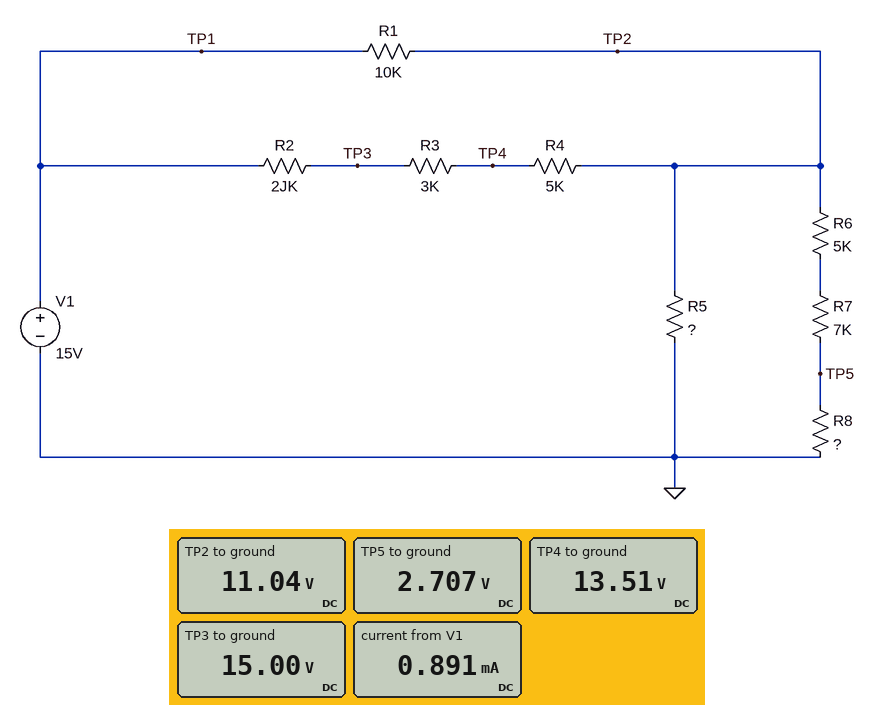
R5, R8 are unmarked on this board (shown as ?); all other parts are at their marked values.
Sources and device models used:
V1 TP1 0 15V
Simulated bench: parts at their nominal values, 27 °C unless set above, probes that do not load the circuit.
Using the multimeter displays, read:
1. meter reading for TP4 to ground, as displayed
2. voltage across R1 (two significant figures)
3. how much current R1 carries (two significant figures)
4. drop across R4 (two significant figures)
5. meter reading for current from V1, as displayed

13.51 V
4.0 V
400 µA
2.5 V
0.891 mA
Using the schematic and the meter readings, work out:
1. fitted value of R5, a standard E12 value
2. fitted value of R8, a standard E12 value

56 kΩ
3.9 kΩ
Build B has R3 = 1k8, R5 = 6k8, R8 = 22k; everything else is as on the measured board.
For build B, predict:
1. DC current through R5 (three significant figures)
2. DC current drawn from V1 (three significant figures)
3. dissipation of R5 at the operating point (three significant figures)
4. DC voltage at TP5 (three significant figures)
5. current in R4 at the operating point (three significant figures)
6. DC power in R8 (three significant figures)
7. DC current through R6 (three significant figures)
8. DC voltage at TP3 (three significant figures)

1.29 mA
1.54 mA
11.3 mW
5.66 V
919 µA
1.46 mW
257 µA
15.0 V
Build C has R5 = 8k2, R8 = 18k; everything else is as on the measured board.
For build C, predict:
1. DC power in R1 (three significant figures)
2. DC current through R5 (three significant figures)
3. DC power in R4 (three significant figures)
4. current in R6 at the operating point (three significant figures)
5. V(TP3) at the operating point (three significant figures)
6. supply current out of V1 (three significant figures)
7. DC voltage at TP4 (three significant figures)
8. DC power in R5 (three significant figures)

3.75 mW
1.08 mA
2.93 mW
296 µA
15.0 V
1.38 mA
12.7 V
9.60 mW
